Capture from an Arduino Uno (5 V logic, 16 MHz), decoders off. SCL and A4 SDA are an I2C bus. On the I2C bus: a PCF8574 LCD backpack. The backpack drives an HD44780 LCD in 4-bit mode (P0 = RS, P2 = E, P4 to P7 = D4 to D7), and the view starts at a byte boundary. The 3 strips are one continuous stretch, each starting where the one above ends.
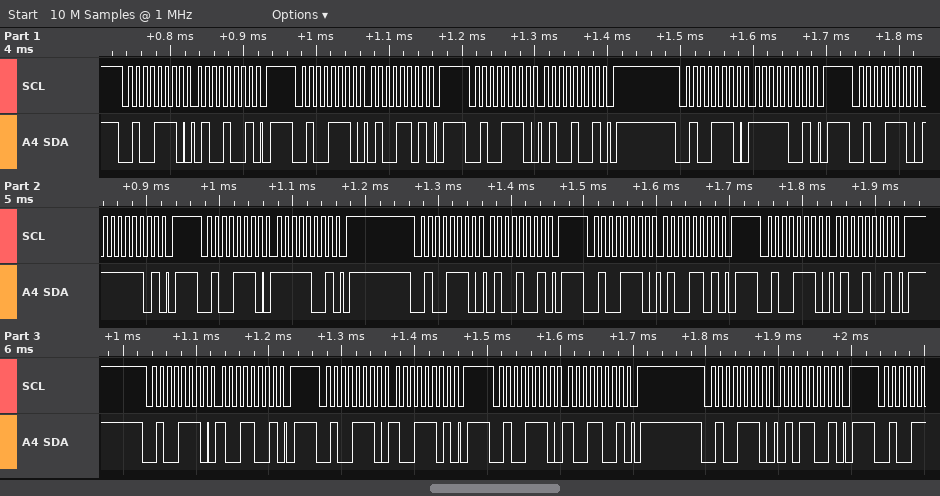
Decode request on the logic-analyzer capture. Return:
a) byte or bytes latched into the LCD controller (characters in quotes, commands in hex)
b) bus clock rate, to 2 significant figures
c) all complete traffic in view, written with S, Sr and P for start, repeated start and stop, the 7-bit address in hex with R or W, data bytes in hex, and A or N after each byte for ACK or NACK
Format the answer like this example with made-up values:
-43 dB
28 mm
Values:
'O' 'I'
100 kHz
S 27W A 49 A P S 27W A 4D A P S 27W A 49 A P S 27W A F9 A P S 27W A FD A P S 27W A F9 A P S 27W A 49 A P S 27W A 4D A P S 27W A 49 A P S 27W A 99 A P S 27W A 9D A P S 27W A 99 A P S 27W A 59 A P
